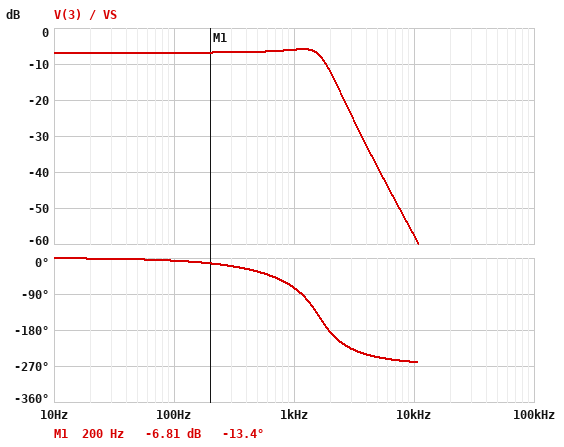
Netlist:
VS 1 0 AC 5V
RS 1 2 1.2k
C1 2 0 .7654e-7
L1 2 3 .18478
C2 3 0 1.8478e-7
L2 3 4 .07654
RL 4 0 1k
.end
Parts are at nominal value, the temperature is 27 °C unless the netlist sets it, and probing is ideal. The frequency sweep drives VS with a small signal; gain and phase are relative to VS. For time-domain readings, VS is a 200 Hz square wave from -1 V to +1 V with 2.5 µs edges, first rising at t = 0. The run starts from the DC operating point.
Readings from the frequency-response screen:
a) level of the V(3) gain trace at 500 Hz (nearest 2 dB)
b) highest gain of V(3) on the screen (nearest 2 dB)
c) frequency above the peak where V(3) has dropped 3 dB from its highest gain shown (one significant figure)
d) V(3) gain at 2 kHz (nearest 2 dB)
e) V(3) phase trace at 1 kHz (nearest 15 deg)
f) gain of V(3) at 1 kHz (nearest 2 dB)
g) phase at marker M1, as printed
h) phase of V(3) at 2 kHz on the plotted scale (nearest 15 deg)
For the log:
-6 dB
-6 dB
2 kHz
-12 dB
-75 deg
-6 dB
-13.4 deg
-180 deg
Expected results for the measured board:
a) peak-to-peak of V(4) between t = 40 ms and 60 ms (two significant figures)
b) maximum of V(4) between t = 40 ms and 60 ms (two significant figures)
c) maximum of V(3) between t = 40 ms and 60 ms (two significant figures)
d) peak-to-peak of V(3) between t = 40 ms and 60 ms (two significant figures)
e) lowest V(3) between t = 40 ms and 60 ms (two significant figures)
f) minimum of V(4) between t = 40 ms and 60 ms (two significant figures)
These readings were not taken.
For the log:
1.1 V
560 mV
610 mV
1.2 V
-610 mV
-560 mV
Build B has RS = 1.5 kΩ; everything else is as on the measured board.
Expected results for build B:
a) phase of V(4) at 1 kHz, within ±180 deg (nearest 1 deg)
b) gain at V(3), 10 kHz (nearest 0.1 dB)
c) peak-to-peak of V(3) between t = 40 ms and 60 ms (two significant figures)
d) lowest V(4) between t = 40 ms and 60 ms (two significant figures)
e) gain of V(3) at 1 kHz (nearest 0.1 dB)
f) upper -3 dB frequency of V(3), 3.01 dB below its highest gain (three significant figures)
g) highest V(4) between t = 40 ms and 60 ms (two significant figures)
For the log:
-99 deg
-59.5 dB
1.1 V
-500 mV
-7.1 dB
1.80 kHz
500 mV
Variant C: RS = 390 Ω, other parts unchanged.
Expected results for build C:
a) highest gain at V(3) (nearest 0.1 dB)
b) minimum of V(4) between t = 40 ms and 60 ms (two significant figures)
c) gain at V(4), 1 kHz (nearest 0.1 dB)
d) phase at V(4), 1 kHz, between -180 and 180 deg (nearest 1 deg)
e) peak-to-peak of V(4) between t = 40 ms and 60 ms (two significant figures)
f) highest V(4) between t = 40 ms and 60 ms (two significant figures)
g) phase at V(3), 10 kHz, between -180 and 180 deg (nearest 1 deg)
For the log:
-2.2 dB
-870 mV
-3.1 dB
-105 deg
1.7 V
870 mV
119 deg
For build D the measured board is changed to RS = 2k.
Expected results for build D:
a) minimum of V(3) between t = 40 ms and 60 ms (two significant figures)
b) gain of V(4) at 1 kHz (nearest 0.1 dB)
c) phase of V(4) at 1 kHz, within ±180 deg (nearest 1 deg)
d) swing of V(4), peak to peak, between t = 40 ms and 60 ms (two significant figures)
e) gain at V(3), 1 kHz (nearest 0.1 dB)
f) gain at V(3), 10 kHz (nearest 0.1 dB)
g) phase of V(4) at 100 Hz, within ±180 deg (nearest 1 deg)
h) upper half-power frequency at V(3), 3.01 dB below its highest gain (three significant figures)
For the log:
-470 mV
-9.6 dB
-98 deg
850 mV
-8.7 dB
-61.9 dB
-9 deg
1.84 kHz
